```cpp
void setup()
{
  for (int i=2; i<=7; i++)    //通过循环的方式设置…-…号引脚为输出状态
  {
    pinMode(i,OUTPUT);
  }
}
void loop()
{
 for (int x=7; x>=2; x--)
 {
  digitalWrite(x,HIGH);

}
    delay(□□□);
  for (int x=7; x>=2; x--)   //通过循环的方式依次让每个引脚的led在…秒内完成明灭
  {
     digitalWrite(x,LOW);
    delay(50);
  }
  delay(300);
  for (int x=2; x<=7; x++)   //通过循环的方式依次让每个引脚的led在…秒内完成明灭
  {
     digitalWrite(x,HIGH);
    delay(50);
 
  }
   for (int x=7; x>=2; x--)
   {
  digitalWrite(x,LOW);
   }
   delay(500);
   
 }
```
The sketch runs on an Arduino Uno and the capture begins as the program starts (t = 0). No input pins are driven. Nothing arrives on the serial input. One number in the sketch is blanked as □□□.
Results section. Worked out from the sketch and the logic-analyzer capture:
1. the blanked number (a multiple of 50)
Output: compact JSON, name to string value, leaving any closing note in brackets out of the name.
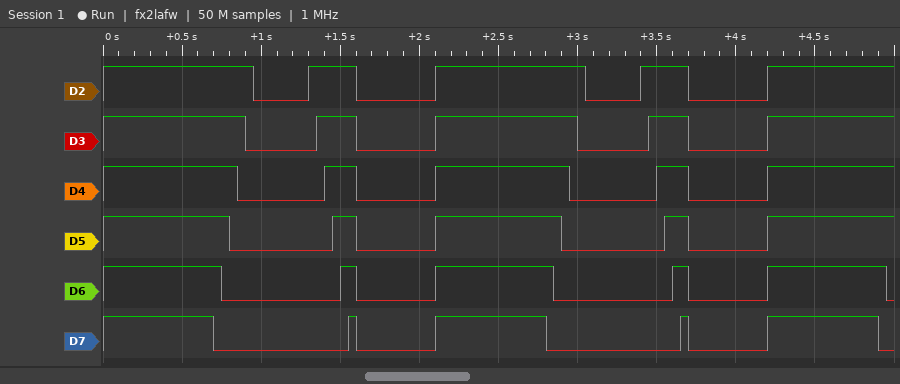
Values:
{"the blanked number": "700"}
